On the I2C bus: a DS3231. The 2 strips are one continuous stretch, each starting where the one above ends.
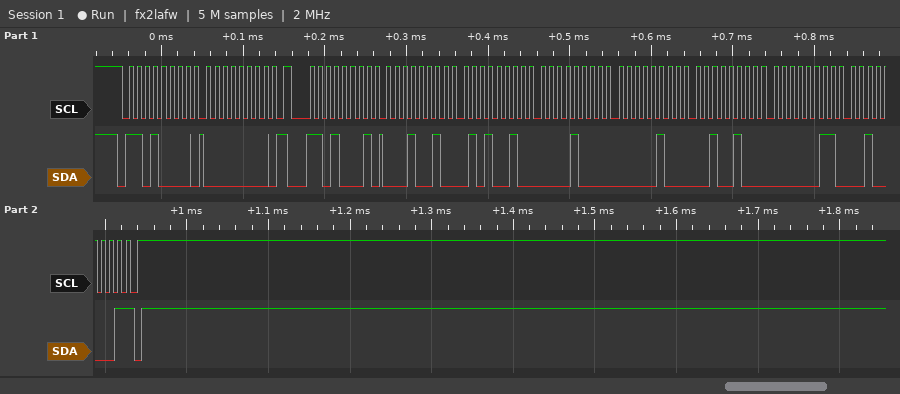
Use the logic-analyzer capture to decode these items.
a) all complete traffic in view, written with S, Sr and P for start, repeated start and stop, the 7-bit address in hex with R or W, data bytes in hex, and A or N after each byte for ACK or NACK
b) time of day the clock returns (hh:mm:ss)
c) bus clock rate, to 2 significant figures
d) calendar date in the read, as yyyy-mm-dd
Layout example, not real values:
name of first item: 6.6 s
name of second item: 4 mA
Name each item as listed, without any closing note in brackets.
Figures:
all complete traffic in view, written with S, Sr and P for start, repeated start and stop, the 7-bit address in hex with R or W, data bytes in hex, and A or N after each byte for ACK or NACK: S 68W A 00 A Sr 68R A 12 A 52 A 08 A 04 A 24 A 03 A 21 N P
time of day the clock returns: 08:52:12
bus clock rate, to 2 significant figures: 100 kHz
calendar date in the read, as yyyy-mm-dd: 2021-03-24
